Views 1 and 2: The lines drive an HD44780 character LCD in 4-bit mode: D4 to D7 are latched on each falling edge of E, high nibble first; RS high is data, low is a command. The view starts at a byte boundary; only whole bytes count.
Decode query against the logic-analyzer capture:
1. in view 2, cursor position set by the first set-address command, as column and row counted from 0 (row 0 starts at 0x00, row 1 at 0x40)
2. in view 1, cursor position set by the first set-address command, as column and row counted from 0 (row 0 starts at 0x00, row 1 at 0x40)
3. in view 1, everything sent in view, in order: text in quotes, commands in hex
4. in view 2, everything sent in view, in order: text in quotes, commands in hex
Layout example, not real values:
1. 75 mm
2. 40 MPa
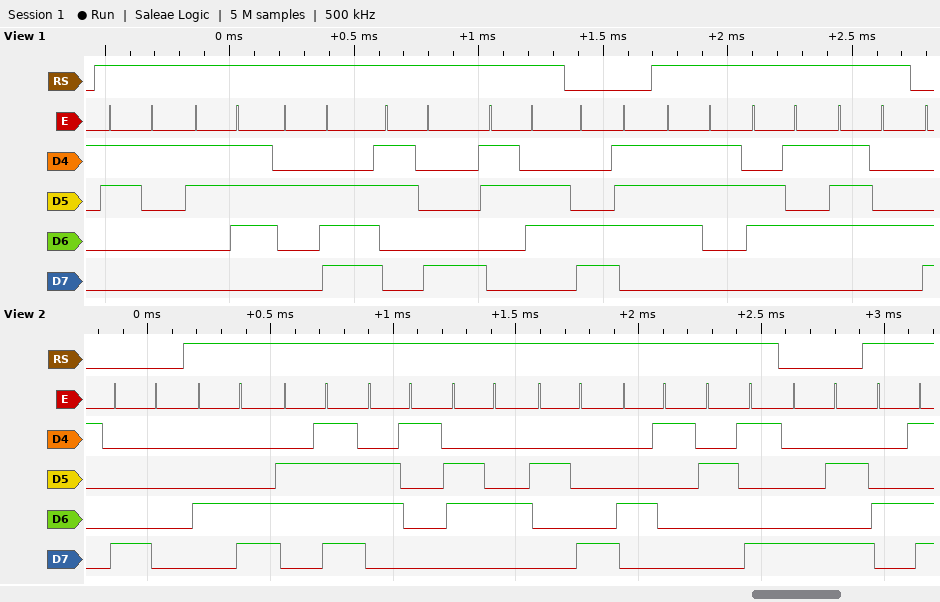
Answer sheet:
1. column 0, row 0
2. column 7, row 1
3. "17.86" 0xC7 "set"
4. 0x80 "Load(A)" 0x8A "M"
